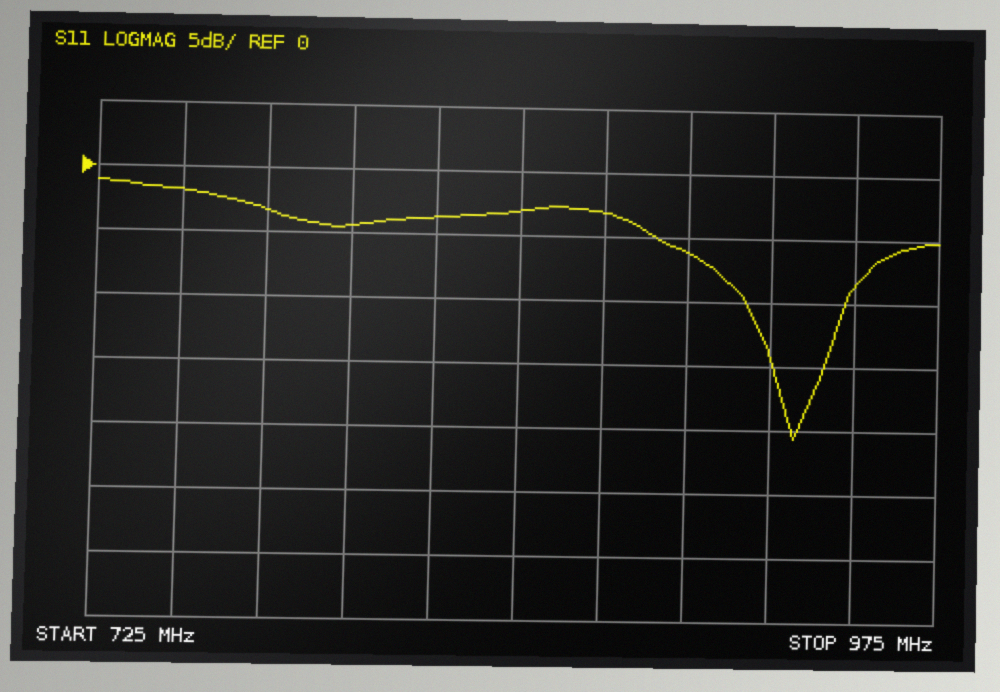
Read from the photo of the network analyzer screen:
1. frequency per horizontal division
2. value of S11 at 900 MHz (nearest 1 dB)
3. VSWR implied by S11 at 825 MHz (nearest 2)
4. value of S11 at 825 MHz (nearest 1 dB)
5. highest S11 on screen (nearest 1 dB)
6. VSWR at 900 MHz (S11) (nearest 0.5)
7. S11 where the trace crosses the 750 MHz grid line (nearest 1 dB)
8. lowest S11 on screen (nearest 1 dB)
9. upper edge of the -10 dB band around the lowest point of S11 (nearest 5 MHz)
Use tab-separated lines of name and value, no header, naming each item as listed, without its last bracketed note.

frequency per horizontal division	25 MHz
value of S11 at 900 MHz	-6 dB
VSWR implied by S11 at 825 MHz	4
value of S11 at 825 MHz	-4 dB
highest S11 on screen	-1 dB
VSWR at 900 MHz (S11)	3.0
S11 where the trace crosses the 750 MHz grid line	-2 dB
lowest S11 on screen	-21 dB
upper edge of the -10 dB band around the lowest point of S11	945 MHz
